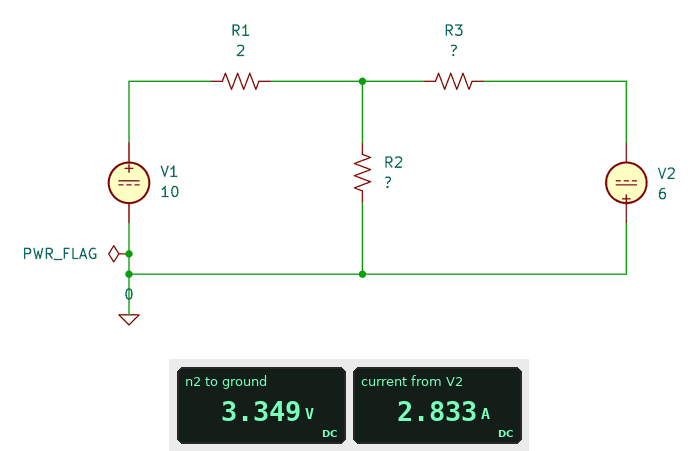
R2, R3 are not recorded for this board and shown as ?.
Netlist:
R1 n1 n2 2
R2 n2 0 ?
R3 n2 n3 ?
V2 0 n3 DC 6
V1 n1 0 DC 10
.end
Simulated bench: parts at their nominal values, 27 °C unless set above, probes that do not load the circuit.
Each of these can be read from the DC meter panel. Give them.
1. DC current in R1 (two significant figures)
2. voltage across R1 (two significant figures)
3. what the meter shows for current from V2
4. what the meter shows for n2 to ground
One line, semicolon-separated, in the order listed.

3.3 A; 6.7 V; 2.833 A; 3.349 V
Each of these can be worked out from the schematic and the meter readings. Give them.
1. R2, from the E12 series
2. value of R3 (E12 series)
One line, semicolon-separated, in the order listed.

6.8 Ω; 3.3 Ω
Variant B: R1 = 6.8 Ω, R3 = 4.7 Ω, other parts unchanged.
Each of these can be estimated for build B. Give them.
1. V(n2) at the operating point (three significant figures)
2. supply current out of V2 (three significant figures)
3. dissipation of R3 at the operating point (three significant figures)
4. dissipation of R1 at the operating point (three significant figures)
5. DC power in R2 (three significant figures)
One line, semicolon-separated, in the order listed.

383 mV; 1.36 A; 8.67 W; 13.6 W; 21.5 mW
